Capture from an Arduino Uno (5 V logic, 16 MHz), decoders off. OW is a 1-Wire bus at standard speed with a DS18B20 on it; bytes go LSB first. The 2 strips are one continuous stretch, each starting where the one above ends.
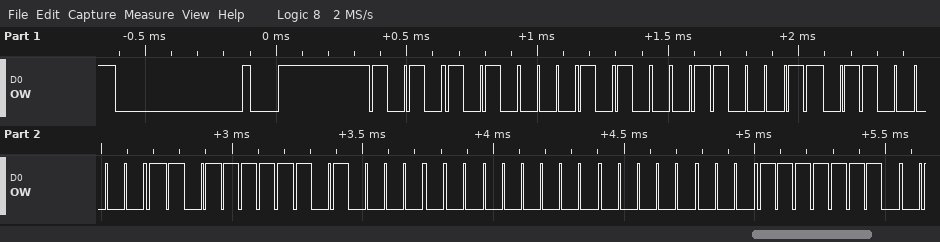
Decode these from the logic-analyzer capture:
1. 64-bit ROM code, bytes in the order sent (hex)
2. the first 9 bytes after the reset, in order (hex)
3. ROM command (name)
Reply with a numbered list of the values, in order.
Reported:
1. 28 C6 06 FB 05 00 00 7F
2. 55 28 C6 06 FB 05 00 00 7F
3. Match ROM
